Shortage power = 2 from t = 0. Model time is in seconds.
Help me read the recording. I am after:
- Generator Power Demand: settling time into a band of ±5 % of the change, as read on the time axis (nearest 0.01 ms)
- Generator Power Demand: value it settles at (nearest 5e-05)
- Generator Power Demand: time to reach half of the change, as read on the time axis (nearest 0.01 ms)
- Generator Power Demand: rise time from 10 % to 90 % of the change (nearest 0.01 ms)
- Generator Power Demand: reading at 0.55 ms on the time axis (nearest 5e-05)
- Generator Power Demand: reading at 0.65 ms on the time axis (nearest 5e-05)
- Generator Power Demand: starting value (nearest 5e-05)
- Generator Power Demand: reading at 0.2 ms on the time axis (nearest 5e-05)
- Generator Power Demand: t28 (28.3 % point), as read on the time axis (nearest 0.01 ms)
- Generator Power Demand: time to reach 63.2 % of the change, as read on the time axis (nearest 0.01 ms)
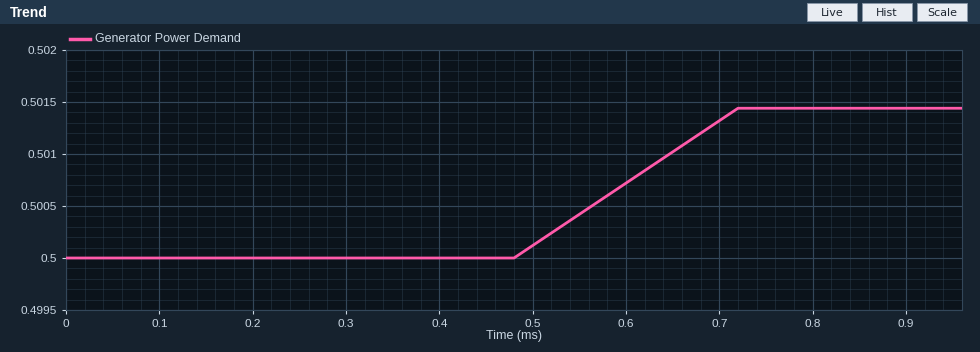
0.71 ms
0.50145
0.60 ms
0.19 ms
0.50040
0.50100
0.50000
0.50000
0.55 ms
0.63 ms
